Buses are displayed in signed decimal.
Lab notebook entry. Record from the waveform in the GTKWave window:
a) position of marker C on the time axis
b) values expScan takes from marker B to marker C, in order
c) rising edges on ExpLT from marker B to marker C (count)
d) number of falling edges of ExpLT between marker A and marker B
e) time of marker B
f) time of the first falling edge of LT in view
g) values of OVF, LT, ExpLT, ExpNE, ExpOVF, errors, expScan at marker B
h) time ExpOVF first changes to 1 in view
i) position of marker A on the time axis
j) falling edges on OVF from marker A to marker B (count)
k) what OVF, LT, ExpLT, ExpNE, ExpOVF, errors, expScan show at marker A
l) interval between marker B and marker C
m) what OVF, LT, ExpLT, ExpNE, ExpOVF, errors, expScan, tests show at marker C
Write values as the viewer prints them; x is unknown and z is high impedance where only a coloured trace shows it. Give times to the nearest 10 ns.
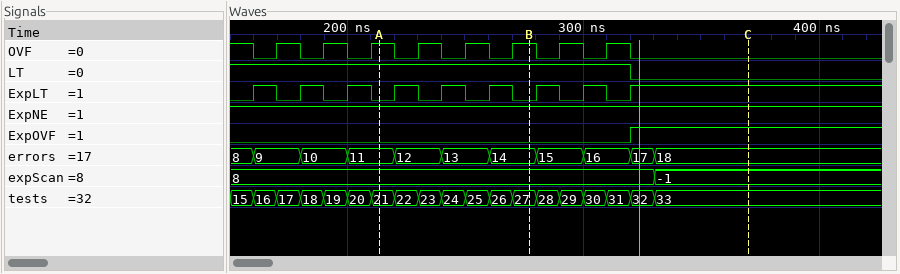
370 ns
8, -1
3
3
280 ns
320 ns
OVF=1, LT=1, ExpLT=0, ExpNE=1, ExpOVF=0, errors=14, expScan=8
320 ns
210 ns
3
OVF=1, LT=1, ExpLT=0, ExpNE=1, ExpOVF=0, errors=11, expScan=8
90 ns
OVF=0, LT=0, ExpLT=1, ExpNE=1, ExpOVF=1, errors=18, expScan=-1, tests=33
